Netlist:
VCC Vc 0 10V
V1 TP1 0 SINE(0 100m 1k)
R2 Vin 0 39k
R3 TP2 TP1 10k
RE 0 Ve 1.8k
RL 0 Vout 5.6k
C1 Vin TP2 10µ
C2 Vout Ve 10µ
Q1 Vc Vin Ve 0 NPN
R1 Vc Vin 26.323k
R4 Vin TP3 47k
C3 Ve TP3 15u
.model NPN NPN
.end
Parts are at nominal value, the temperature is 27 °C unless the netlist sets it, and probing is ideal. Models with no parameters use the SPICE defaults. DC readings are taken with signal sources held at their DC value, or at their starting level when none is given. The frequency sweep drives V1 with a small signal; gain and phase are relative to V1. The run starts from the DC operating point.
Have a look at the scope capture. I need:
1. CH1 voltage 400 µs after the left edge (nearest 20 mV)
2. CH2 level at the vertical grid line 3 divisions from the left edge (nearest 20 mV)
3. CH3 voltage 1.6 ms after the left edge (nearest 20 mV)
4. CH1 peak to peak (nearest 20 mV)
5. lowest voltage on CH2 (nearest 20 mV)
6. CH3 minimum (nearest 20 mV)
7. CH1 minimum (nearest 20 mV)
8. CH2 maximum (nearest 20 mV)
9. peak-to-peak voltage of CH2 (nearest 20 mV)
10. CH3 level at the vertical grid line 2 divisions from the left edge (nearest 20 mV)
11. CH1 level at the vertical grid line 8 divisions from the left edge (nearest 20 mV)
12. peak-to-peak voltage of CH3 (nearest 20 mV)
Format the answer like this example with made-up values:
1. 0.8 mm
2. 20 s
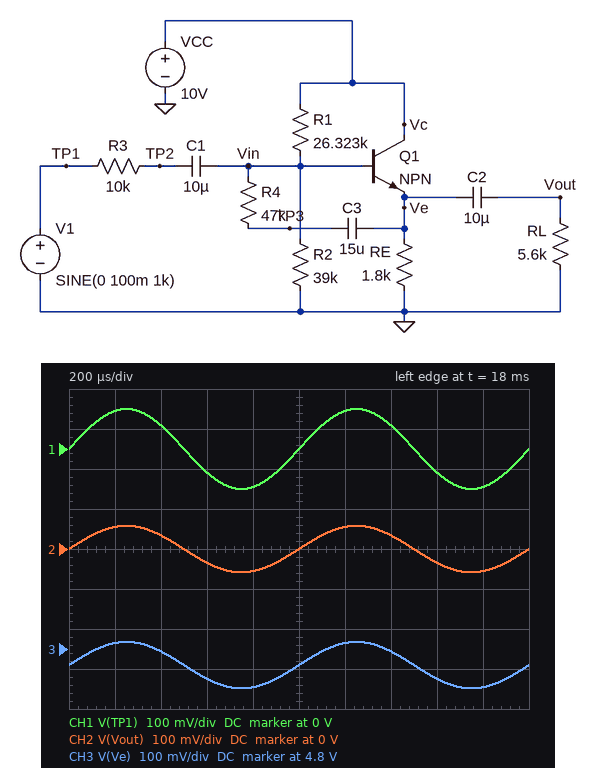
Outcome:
1. 60 mV
2. -40 mV
3. 4.72 V
4. 200 mV
5. -60 mV
6. 4.70 V
7. -100 mV
8. 60 mV
9. 120 mV
10. 4.80 V
11. -60 mV
12. 120 mV
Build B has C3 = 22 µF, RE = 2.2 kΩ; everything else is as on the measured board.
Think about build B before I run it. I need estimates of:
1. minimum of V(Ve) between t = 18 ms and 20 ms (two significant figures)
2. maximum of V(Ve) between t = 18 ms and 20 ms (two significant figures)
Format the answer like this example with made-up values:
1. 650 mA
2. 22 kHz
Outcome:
1. 4.8 V
2. 4.9 V
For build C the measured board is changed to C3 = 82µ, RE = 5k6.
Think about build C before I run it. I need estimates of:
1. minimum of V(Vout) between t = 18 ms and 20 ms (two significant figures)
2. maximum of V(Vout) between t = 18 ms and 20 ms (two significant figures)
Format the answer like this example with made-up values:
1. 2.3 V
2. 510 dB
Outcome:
1. -59 mV
2. 59 mV
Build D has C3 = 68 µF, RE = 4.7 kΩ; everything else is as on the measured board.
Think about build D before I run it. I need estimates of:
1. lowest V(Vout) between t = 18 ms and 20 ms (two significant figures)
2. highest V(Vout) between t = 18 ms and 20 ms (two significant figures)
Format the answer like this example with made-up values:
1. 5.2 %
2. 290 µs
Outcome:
1. -59 mV
2. 59 mV
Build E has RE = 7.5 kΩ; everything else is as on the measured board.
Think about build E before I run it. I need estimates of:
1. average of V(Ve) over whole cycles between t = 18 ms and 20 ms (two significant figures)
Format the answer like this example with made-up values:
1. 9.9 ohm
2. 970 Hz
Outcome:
1. 5.1 V
